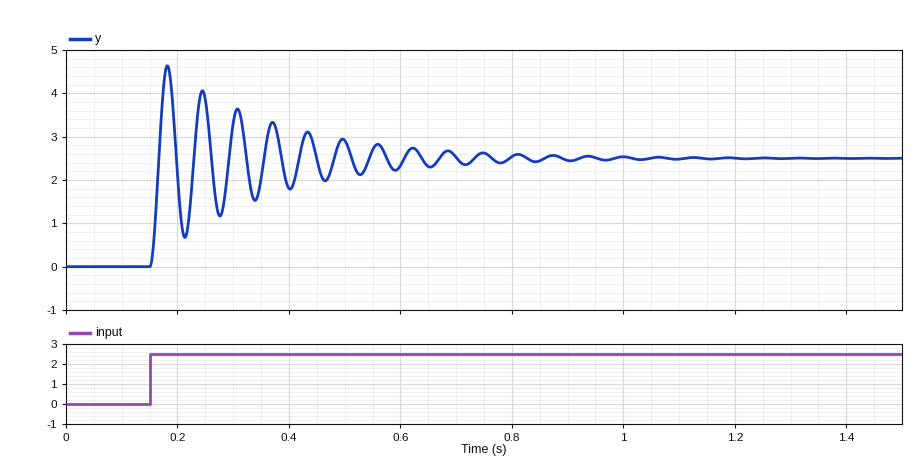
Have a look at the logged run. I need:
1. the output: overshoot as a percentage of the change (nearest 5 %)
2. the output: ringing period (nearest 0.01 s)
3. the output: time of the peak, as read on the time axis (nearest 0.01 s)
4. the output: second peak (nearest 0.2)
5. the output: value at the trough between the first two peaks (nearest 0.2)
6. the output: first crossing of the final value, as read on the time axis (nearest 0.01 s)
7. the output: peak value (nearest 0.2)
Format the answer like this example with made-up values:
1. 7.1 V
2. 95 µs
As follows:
1. 85 %
2. 0.06 s
3. 0.18 s
4. 4.0
5. 0.6
6. 0.17 s
7. 4.6
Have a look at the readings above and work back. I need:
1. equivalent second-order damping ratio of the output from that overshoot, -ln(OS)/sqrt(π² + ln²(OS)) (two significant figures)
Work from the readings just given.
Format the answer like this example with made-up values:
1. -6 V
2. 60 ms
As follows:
1. 0.052
